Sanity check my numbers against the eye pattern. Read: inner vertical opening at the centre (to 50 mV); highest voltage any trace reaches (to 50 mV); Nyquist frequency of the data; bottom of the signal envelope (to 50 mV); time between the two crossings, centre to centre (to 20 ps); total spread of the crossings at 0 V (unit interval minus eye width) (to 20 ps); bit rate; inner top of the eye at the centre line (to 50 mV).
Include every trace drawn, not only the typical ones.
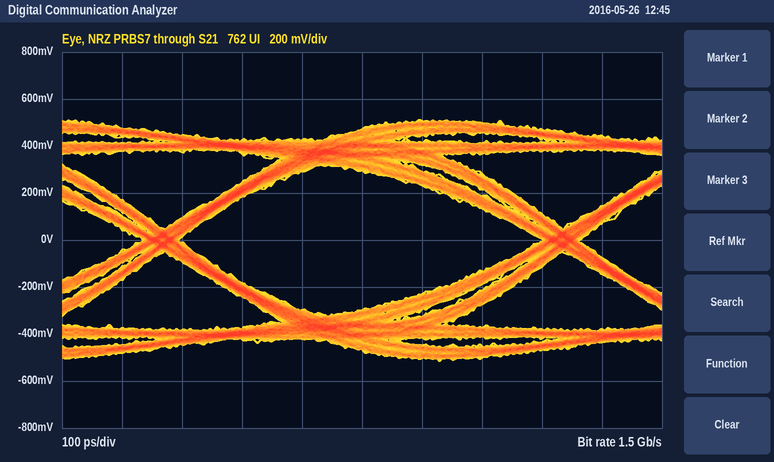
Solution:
600 mV
500 mV
750 MHz
-500 mV
660 ps
60 ps
1.5 Gb/s
300 mV
